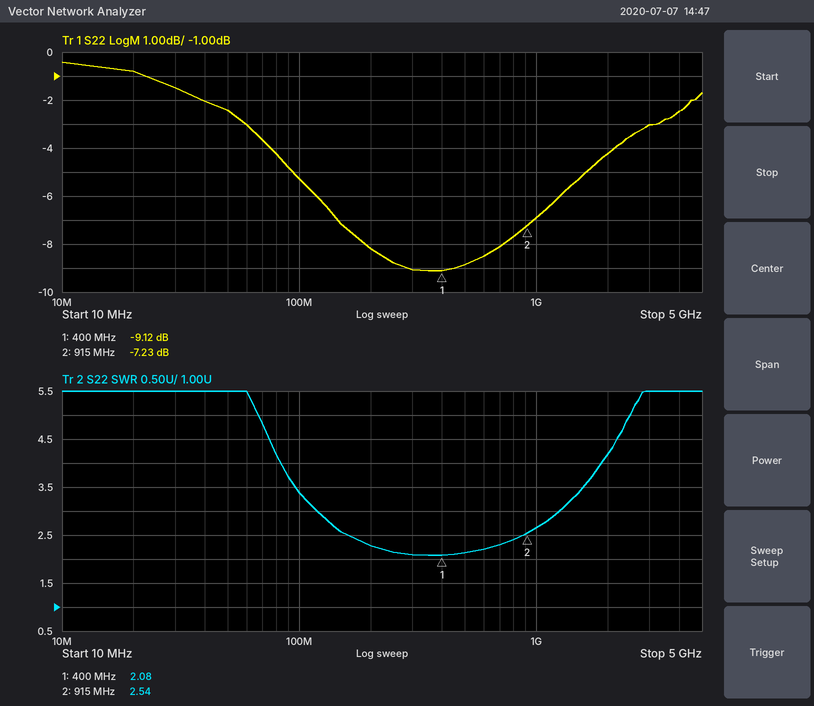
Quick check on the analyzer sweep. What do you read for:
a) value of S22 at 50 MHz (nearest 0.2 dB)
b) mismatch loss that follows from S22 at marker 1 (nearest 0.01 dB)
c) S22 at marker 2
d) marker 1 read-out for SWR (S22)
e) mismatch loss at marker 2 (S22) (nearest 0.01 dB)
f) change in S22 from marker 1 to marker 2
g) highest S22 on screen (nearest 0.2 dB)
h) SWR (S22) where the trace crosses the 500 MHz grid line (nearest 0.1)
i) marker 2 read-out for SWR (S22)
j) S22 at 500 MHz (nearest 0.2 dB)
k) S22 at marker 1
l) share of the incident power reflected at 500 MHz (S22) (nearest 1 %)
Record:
-2.4 dB
0.57 dB
-7.23 dB
2.08
0.91 dB
1.89 dB
-0.4 dB
2.1
2.54
-8.8 dB
-9.12 dB
13 %
